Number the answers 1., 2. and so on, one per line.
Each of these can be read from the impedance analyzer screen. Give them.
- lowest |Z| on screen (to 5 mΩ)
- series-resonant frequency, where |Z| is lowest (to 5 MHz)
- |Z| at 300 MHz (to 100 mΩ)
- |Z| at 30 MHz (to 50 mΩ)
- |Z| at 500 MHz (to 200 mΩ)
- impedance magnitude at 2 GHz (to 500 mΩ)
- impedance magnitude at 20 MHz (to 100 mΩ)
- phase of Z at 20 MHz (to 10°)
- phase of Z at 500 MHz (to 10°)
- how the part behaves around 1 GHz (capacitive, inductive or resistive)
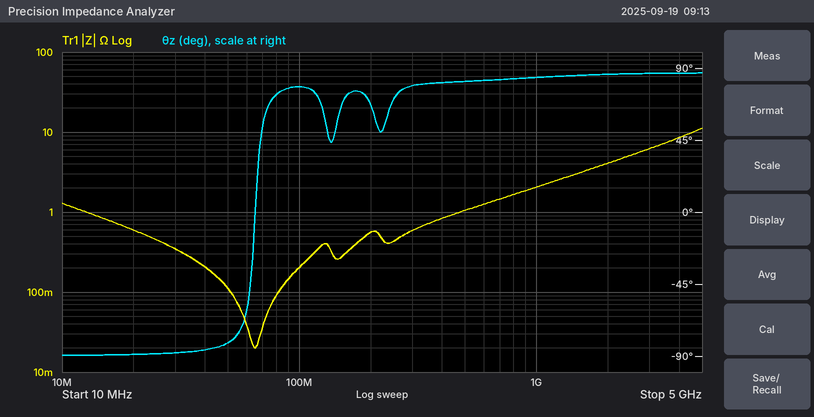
1. 20 mΩ
2. 65 MHz
3. 600 mΩ
4. 350 mΩ
5. 1.0 Ω
6. 4.0 Ω
7. 600 mΩ
8. -90°
9. 80°
10. inductive
